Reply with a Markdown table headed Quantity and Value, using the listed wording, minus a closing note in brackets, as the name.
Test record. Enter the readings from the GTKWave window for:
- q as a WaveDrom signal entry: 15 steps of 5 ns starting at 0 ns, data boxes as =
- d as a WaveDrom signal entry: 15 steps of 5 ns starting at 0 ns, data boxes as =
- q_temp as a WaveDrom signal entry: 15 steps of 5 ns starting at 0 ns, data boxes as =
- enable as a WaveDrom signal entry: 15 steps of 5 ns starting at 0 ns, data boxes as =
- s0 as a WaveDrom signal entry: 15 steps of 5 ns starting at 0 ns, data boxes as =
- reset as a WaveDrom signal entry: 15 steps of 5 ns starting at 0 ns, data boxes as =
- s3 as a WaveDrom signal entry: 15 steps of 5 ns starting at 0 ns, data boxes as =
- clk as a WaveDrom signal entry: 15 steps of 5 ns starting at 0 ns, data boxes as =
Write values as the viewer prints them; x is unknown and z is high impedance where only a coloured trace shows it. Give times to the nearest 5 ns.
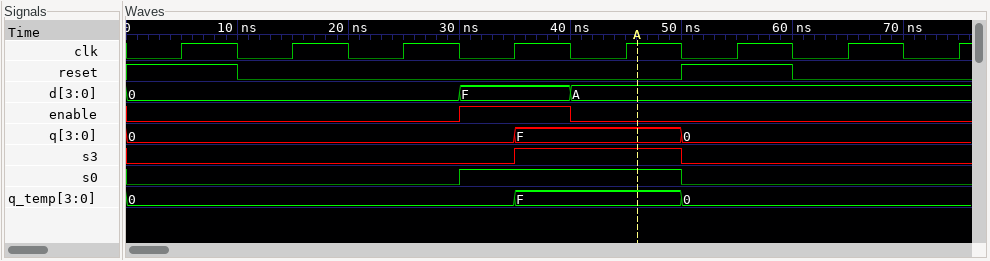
| Quantity | Value |
|---|---|
| q as a WaveDrom signal entry: 15 steps of 5 ns starting at 0 ns, data boxes as = | {name: 'q', wave: '=......=..=....', data: '0 F 0'} |
| d as a WaveDrom signal entry: 15 steps of 5 ns starting at 0 ns, data boxes as = | {name: 'd', wave: '=.....=.=......', data: '0 F A'} |
| q_temp as a WaveDrom signal entry: 15 steps of 5 ns starting at 0 ns, data boxes as = | {name: 'q_temp', wave: '=......=..=....', data: '0 F 0'} |
| enable as a WaveDrom signal entry: 15 steps of 5 ns starting at 0 ns, data boxes as = | {name: 'enable', wave: '0.....1.0......'} |
| s0 as a WaveDrom signal entry: 15 steps of 5 ns starting at 0 ns, data boxes as = | {name: 's0', wave: '0.....1...0....'} |
| reset as a WaveDrom signal entry: 15 steps of 5 ns starting at 0 ns, data boxes as = | {name: 'reset', wave: '1.0.......1.0..'} |
| s3 as a WaveDrom signal entry: 15 steps of 5 ns starting at 0 ns, data boxes as = | {name: 's3', wave: '0......1..0....'} |
| clk as a WaveDrom signal entry: 15 steps of 5 ns starting at 0 ns, data boxes as = | {name: 'clk', wave: '010101010101010'} |
